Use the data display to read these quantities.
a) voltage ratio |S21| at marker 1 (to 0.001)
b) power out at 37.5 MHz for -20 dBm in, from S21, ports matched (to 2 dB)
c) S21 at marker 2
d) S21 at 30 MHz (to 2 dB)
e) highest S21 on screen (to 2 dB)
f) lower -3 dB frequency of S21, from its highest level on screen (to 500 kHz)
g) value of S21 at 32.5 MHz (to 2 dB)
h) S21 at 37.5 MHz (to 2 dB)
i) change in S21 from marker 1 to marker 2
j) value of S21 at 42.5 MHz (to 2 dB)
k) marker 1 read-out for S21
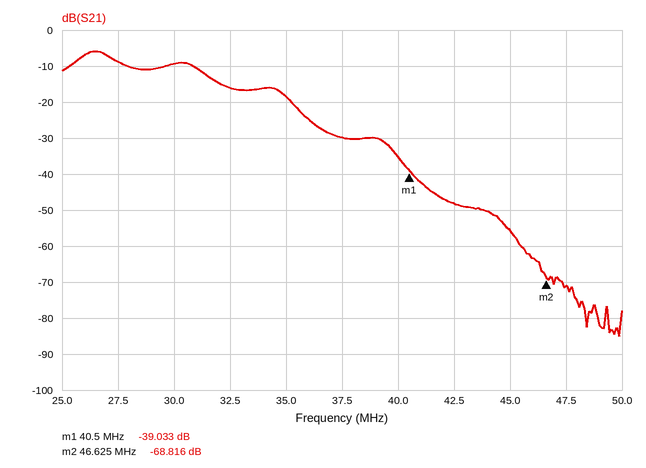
0.011
-50 dBm
-68.816 dB
-10 dB
-6 dB
25.5 MHz
-16 dB
-30 dB
-29.783 dB
-48 dB
-39.033 dB
